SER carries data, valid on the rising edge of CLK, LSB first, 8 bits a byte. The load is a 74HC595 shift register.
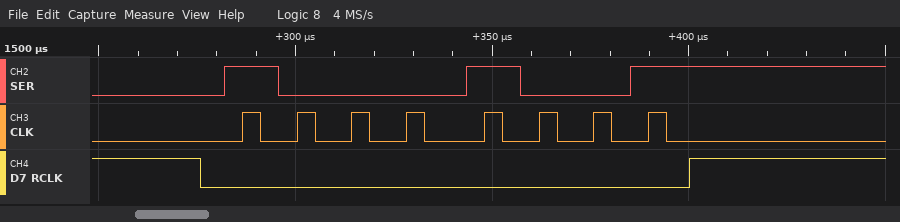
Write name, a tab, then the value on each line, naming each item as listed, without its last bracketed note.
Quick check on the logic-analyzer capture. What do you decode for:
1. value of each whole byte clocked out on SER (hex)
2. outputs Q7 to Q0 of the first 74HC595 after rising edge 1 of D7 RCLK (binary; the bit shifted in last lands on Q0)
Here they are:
value of each whole byte clocked out on SER	0x91
outputs Q7 to Q0 of the first 74HC595 after rising edge 1 of D7 RCLK	10001001
